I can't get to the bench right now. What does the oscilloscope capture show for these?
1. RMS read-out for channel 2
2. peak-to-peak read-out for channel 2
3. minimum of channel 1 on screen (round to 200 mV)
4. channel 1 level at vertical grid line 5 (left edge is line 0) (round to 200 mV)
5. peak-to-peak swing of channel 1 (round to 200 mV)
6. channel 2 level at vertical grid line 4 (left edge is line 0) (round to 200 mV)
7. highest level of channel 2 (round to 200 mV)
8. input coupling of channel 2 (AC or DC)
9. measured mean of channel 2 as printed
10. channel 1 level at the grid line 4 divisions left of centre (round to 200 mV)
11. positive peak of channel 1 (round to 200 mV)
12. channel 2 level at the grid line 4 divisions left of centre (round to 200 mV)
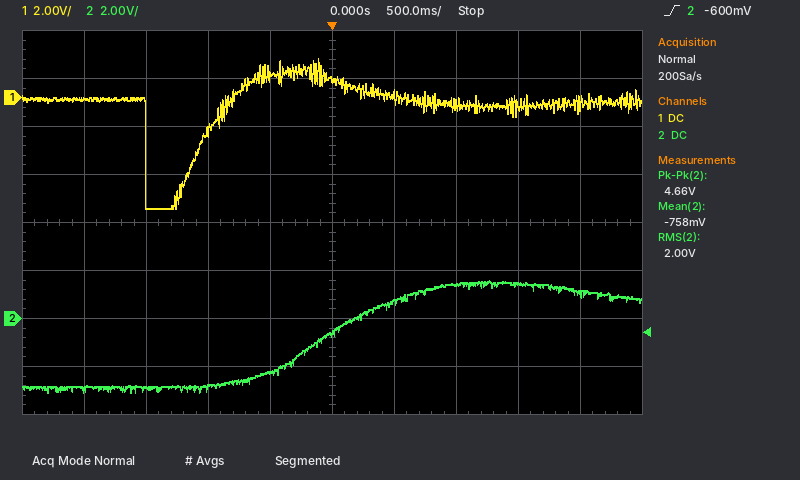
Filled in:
2.00 V
4.66 V
-4.6 V
800 mV
6.2 V
-2.2 V
1.6 V
DC
-758 mV
0.0 V
1.6 V
-3.0 V
